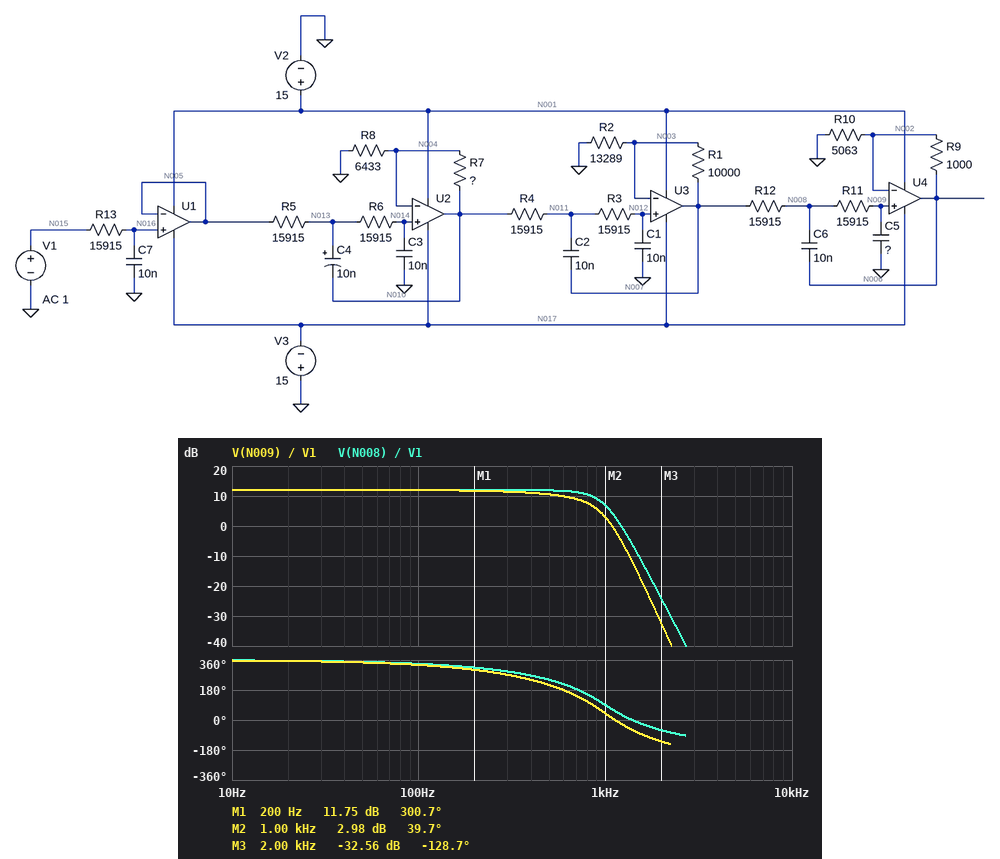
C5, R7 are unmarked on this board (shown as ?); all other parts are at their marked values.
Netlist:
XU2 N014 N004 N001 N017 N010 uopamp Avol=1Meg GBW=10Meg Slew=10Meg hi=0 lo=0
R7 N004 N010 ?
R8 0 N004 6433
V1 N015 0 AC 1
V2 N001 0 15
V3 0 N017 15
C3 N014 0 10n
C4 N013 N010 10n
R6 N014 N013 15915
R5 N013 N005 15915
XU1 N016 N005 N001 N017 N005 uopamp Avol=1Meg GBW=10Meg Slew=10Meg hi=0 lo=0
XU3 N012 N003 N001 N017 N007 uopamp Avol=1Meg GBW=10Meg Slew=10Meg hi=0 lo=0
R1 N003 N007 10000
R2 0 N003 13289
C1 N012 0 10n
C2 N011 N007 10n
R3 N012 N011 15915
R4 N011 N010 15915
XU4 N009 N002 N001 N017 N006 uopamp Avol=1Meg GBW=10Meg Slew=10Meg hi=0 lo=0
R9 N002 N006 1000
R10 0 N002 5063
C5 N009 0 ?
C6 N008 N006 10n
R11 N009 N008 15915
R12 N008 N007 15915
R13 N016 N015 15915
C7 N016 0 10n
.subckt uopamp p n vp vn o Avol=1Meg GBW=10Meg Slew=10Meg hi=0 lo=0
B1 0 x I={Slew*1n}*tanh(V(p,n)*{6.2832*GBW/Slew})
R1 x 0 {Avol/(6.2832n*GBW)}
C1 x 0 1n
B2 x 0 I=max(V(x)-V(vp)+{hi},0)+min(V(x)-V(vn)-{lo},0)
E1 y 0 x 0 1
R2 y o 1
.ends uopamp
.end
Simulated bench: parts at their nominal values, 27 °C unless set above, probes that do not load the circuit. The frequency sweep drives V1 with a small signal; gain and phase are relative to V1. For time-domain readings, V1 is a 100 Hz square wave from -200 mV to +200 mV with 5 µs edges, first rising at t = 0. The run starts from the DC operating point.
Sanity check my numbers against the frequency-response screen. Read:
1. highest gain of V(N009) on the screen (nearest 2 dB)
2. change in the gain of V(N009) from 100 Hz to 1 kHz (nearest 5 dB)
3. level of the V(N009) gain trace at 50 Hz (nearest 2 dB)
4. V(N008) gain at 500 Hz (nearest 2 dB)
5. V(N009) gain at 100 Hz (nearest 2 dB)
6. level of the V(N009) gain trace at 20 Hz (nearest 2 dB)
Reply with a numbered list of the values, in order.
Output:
1. 12 dB
2. -10 dB
3. 12 dB
4. 12 dB
5. 12 dB
6. 12 dB
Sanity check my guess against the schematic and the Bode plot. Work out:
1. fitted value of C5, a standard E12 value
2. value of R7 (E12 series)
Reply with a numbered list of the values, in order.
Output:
1. 12 nF
2. 8.2 kΩ
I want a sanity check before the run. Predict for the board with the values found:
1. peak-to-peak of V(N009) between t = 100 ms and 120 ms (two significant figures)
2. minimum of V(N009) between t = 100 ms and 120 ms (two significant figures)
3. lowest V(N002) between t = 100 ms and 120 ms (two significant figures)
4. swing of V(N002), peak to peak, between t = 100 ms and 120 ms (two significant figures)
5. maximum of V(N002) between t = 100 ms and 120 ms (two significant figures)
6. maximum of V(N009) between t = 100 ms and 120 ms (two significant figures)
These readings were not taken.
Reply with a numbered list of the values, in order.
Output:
1. 1.7 V
2. -870 mV
3. -870 mV
4. 1.7 V
5. 870 mV
6. 870 mV
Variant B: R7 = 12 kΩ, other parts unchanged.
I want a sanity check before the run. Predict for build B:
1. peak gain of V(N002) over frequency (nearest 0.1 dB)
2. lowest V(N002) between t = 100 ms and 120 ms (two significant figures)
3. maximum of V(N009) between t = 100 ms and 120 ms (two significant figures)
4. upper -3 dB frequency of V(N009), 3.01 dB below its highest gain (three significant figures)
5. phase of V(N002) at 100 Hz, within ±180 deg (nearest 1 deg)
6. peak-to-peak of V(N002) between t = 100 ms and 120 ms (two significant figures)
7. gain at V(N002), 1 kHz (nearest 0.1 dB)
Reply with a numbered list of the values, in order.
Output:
1. 19.9 dB
2. -1.3 V
3. 1.3 V
4. 1.04 kHz
5. -26 deg
6. 2.6 V
7. 19.6 dB
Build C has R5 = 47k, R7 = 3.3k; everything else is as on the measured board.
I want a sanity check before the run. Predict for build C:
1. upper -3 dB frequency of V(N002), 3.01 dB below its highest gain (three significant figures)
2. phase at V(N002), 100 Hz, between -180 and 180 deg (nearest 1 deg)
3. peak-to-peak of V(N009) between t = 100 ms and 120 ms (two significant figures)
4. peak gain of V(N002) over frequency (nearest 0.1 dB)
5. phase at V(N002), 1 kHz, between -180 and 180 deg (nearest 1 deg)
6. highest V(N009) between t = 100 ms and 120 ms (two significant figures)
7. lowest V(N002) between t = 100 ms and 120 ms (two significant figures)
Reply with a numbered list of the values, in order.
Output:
1. 407 Hz
2. -40 deg
3. 1.1 V
4. 8.5 dB
5. 1 deg
6. 550 mV
7. -550 mV
